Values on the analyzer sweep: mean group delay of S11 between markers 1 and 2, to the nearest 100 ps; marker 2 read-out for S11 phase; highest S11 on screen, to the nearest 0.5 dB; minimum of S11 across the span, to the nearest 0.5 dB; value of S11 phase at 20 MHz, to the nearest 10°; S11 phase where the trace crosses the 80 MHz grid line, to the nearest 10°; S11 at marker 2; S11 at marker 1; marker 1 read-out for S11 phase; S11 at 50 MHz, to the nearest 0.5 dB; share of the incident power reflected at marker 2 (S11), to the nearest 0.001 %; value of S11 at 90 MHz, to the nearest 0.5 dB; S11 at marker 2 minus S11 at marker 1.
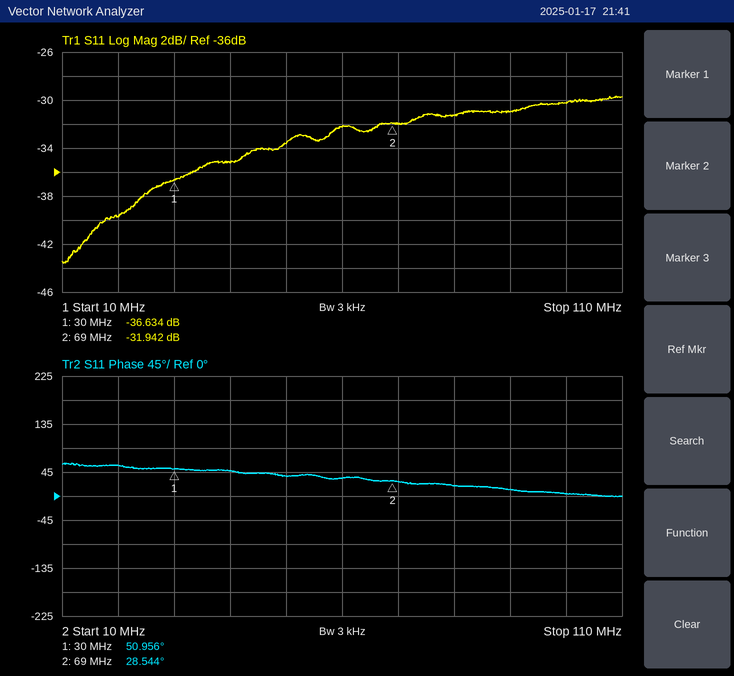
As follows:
1.6 ns
28.544°
-29.5 dB
-43.5 dB
60°
20°
-31.942 dB
-36.634 dB
50.956°
-33.5 dB
0.064 %
-31.0 dB
4.692 dB
